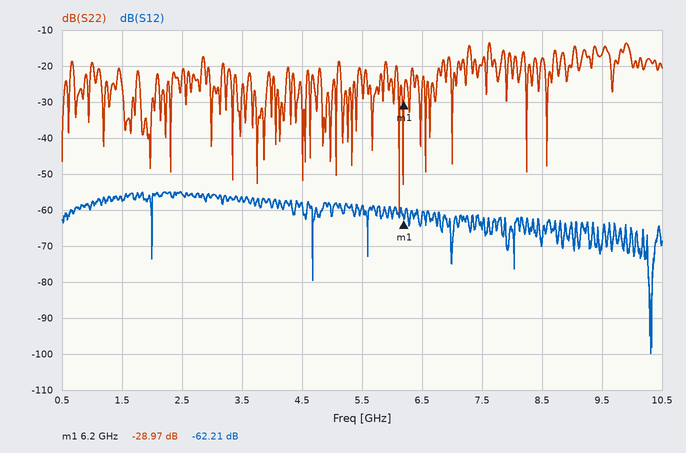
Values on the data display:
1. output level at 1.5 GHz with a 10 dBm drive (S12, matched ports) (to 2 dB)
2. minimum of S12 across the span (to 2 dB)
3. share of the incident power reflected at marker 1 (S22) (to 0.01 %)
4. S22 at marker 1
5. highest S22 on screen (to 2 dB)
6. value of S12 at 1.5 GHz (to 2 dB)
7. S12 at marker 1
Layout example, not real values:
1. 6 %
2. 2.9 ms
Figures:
1. -48 dBm
2. -100 dB
3. 0.13 %
4. -28.97 dB
5. -14 dB
6. -58 dB
7. -62.21 dB
